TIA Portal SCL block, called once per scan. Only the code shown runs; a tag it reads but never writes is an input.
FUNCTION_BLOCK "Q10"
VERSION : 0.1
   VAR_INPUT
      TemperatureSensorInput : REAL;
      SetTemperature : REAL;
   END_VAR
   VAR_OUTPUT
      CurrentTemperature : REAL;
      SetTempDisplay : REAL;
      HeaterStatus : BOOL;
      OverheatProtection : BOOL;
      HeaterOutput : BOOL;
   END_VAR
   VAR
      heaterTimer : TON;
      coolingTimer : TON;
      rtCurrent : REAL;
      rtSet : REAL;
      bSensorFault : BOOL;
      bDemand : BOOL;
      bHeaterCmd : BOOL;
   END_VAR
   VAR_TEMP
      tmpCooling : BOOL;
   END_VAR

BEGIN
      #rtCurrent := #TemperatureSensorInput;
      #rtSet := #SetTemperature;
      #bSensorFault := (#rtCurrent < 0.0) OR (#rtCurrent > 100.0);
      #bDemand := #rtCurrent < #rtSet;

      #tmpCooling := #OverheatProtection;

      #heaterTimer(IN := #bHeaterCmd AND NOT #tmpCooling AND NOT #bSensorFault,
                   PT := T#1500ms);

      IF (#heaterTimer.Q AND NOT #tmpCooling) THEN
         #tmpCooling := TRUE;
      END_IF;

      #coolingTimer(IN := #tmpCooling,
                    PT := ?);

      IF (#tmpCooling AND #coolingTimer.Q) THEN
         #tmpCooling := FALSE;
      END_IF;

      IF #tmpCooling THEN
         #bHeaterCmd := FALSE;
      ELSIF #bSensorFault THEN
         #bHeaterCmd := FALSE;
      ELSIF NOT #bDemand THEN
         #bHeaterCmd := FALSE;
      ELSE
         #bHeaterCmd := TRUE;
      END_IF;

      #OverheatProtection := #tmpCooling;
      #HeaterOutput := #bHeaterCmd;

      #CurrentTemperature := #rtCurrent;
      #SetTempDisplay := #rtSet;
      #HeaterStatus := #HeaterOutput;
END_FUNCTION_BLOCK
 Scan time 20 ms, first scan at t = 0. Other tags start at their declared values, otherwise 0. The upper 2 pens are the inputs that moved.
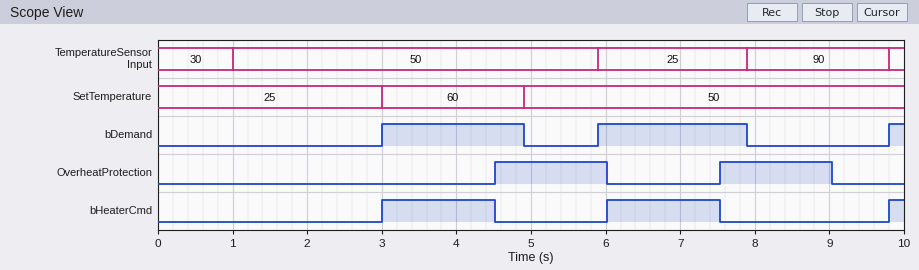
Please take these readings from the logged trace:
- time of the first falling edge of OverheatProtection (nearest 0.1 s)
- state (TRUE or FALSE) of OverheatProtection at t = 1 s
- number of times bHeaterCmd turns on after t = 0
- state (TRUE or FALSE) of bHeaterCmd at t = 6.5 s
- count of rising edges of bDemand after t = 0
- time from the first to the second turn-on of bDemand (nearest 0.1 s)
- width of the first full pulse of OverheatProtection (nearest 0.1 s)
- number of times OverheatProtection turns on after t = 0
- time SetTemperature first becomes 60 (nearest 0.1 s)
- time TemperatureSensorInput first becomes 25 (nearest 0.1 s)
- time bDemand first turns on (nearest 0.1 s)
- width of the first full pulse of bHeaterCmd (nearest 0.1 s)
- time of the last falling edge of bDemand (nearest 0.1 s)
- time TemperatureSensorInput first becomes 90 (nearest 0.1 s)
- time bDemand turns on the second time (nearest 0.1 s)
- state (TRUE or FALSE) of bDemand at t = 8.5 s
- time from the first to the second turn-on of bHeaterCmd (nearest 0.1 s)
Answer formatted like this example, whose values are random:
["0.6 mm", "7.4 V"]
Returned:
["6.0 s", "FALSE", "3", "TRUE", "3", "2.9 s", "1.5 s", "2", "3.0 s", "5.9 s", "3.0 s", "1.5 s", "7.9 s", "7.9 s", "5.9 s", "FALSE", "3.0 s"]
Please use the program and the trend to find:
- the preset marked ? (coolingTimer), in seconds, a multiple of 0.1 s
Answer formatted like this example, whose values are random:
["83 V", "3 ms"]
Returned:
["1.5 s"]
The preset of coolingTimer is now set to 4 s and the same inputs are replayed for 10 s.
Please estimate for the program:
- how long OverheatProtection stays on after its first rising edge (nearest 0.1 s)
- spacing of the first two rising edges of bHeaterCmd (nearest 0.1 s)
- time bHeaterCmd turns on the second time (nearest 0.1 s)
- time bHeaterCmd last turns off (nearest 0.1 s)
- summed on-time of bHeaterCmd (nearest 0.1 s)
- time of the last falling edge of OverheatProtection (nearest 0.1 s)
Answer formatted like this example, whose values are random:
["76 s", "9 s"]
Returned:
["4.0 s", "6.8 s", "9.8 s", "4.5 s", "1.7 s", "8.5 s"]
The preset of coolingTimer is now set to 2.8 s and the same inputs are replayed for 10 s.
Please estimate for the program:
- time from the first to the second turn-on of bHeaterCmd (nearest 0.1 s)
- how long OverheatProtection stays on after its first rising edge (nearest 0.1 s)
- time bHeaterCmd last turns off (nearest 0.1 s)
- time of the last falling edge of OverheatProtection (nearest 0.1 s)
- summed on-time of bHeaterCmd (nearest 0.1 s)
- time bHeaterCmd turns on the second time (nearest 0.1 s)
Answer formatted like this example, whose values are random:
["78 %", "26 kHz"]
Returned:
["4.3 s", "2.8 s", "7.9 s", "7.3 s", "2.3 s", "7.3 s"]
